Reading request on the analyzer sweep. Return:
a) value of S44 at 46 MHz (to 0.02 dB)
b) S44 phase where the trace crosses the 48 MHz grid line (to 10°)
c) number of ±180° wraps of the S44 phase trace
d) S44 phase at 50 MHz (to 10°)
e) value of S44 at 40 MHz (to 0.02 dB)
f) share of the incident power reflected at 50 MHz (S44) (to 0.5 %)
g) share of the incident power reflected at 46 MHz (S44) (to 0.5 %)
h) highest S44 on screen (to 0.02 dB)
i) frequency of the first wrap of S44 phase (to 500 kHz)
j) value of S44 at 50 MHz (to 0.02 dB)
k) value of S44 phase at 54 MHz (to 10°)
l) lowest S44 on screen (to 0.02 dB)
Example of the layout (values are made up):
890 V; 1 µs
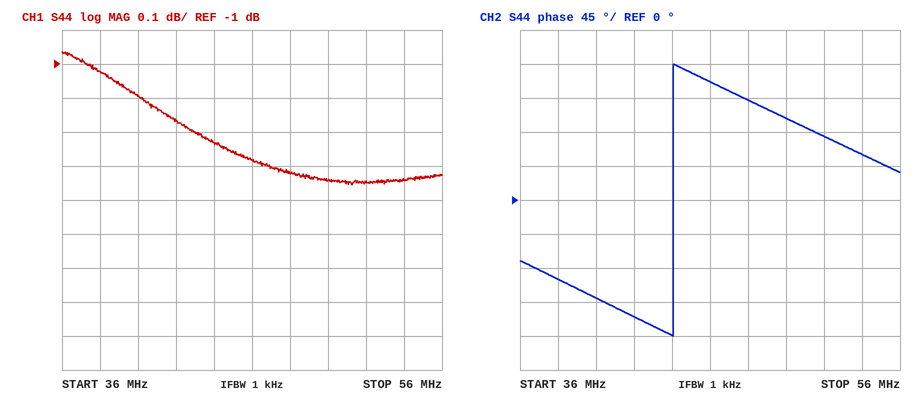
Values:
-1.28 dB; 130°; 1; 110°; -1.10 dB; 73.5 %; 74.5 %; -0.96 dB; 44.0 MHz; -1.34 dB; 60°; -1.36 dB
